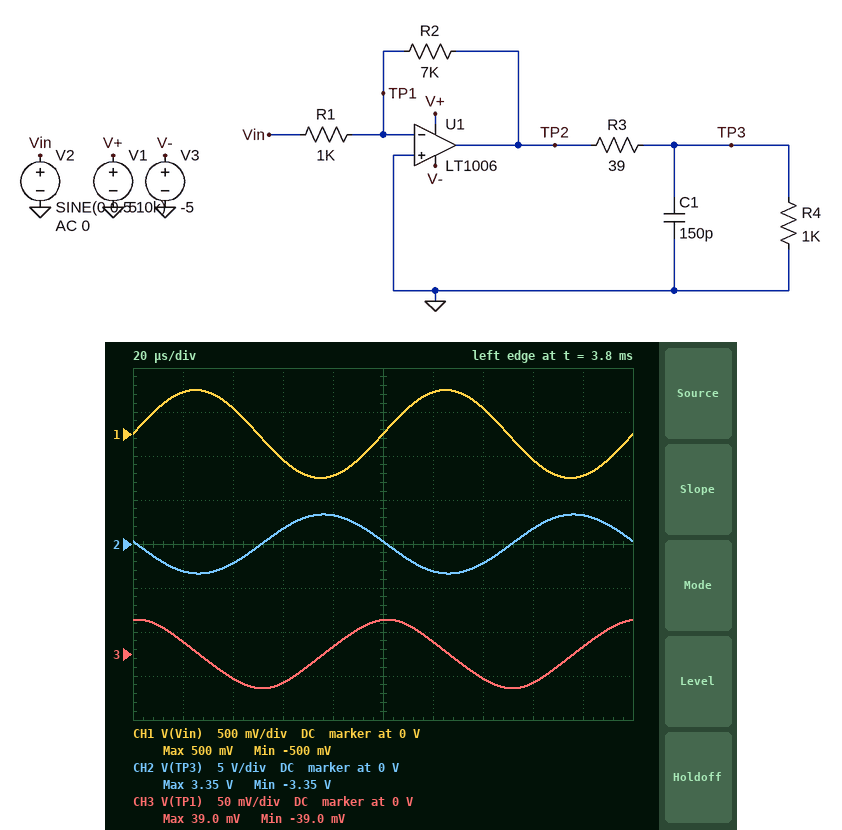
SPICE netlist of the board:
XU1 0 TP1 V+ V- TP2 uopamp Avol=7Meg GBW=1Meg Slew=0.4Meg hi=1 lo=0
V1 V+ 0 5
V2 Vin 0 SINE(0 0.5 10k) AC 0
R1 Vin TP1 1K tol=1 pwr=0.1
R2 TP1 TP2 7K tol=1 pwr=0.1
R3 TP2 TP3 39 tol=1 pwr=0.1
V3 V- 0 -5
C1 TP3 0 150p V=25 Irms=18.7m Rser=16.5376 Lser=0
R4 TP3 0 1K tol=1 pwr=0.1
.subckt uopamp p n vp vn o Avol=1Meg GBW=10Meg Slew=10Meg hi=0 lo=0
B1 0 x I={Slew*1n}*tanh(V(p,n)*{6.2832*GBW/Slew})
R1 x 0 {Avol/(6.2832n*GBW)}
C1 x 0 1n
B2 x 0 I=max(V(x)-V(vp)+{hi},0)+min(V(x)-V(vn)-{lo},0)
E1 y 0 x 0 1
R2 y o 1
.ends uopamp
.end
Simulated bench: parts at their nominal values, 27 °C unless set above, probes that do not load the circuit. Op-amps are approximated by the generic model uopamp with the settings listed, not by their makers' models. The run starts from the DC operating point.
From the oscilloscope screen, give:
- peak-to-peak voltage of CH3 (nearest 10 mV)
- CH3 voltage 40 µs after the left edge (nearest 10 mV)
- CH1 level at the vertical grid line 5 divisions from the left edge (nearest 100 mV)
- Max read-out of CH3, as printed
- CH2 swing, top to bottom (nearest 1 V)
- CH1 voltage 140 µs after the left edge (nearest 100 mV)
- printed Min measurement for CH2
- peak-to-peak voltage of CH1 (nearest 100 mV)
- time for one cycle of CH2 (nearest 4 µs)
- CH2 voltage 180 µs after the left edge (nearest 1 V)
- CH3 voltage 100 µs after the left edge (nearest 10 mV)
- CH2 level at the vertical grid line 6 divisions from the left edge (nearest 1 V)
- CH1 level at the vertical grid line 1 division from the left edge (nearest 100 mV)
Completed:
80 mV
-30 mV
0 V
39.0 mV
7 V
300 mV
-3.35 V
1.0 V
100 µs
3 V
40 mV
-3 V
500 mV
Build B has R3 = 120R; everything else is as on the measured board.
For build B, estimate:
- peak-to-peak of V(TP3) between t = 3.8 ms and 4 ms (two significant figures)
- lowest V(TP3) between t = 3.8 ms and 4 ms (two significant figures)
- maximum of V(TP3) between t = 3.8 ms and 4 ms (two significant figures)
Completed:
6.2 V
-3.1 V
3.1 V
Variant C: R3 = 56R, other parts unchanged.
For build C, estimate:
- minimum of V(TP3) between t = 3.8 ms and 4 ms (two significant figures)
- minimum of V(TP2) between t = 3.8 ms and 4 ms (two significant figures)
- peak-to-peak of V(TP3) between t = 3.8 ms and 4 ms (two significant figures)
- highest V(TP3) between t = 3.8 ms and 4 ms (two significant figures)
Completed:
-3.3 V
-3.5 V
6.6 V
3.3 V
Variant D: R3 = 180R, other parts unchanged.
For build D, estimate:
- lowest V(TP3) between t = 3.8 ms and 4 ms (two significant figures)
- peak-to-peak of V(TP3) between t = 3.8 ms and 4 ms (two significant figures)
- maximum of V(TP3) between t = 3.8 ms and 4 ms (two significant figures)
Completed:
-3.0 V
5.9 V
3.0 V
